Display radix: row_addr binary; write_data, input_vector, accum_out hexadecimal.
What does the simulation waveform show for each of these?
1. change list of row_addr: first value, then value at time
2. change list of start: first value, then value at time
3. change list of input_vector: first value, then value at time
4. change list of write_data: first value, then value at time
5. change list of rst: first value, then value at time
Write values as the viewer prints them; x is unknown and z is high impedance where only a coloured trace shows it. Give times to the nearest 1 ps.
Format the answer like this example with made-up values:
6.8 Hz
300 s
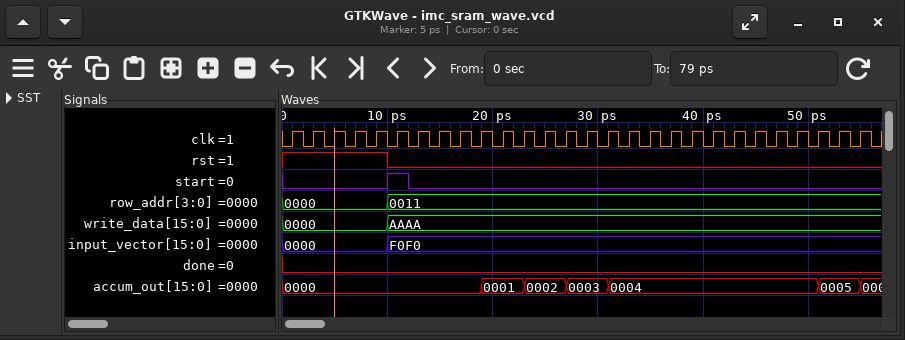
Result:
0000, 0011 at 10 ps
0, 1 at 10 ps, 0 at 12 ps
0000, F0F0 at 10 ps
0000, AAAA at 10 ps
1, 0 at 10 ps
